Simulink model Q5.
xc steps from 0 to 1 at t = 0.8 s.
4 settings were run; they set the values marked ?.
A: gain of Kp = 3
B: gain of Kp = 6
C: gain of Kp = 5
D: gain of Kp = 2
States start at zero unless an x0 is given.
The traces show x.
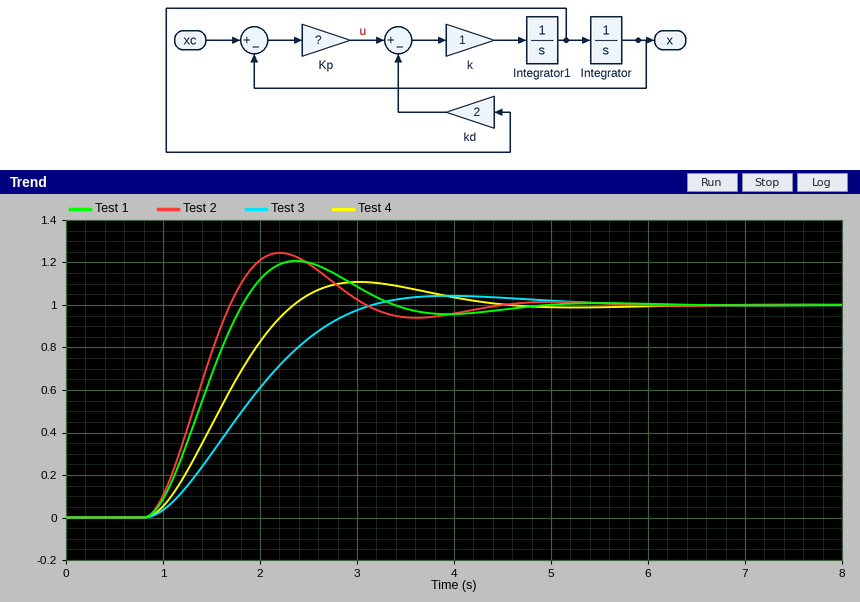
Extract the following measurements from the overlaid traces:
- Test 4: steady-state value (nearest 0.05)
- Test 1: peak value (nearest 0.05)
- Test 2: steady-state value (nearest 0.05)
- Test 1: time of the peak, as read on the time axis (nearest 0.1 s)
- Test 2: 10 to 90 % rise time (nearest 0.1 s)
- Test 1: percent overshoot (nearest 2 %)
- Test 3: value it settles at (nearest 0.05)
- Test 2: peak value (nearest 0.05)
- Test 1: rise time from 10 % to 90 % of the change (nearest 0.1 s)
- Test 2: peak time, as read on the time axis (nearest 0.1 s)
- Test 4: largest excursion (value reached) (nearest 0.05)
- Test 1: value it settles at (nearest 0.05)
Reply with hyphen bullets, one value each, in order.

- 1.00
- 1.20
- 1.00
- 2.4 s
- 0.6 s
- 20 %
- 1.00
- 1.25
- 0.7 s
- 2.2 s
- 1.10
- 1.00
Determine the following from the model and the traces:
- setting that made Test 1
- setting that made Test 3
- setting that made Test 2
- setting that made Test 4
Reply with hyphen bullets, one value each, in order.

- C
- D
- B
- A
